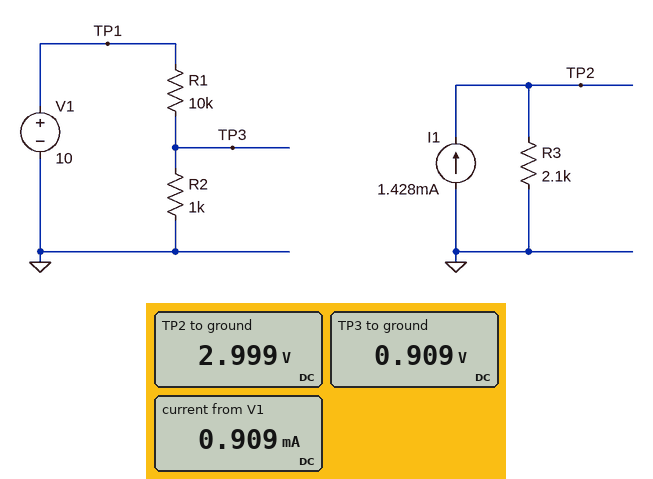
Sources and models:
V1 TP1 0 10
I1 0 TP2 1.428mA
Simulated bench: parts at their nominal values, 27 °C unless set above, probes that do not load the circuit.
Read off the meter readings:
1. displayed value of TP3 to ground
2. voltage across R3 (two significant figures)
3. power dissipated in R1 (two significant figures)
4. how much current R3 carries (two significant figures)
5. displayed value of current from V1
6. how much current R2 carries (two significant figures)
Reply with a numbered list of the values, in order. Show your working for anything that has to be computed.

1. 0.909 V
2. 2.999 V = 3.0 V
3. (10 V - 909 mV)^2 / 10 kΩ = 8.3 mW
4. (2.999 V) / 2.1 kΩ = 1.4 mA
5. 0.909 mA
6. (909 mV) / 1 kΩ = 910 µA
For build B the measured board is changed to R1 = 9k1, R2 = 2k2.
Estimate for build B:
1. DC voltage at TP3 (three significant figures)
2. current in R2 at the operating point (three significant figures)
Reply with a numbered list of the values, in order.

1. 1.95 V
2. 885 µA
